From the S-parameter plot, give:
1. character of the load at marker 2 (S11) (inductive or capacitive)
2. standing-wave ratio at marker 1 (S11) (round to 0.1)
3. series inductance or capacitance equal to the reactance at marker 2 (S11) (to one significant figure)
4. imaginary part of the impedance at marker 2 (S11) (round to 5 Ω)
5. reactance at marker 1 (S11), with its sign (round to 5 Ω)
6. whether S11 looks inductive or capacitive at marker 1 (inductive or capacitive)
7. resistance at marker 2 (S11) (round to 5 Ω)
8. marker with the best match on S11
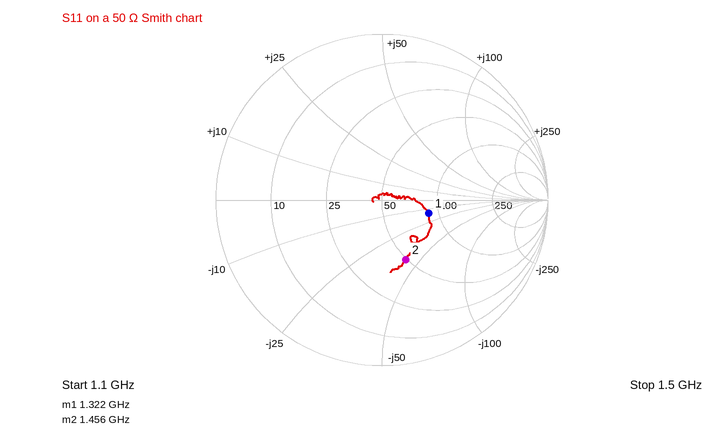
capacitive
1.8
3 pF
-40 Ω
-15 Ω
capacitive
50 Ω
marker 1
